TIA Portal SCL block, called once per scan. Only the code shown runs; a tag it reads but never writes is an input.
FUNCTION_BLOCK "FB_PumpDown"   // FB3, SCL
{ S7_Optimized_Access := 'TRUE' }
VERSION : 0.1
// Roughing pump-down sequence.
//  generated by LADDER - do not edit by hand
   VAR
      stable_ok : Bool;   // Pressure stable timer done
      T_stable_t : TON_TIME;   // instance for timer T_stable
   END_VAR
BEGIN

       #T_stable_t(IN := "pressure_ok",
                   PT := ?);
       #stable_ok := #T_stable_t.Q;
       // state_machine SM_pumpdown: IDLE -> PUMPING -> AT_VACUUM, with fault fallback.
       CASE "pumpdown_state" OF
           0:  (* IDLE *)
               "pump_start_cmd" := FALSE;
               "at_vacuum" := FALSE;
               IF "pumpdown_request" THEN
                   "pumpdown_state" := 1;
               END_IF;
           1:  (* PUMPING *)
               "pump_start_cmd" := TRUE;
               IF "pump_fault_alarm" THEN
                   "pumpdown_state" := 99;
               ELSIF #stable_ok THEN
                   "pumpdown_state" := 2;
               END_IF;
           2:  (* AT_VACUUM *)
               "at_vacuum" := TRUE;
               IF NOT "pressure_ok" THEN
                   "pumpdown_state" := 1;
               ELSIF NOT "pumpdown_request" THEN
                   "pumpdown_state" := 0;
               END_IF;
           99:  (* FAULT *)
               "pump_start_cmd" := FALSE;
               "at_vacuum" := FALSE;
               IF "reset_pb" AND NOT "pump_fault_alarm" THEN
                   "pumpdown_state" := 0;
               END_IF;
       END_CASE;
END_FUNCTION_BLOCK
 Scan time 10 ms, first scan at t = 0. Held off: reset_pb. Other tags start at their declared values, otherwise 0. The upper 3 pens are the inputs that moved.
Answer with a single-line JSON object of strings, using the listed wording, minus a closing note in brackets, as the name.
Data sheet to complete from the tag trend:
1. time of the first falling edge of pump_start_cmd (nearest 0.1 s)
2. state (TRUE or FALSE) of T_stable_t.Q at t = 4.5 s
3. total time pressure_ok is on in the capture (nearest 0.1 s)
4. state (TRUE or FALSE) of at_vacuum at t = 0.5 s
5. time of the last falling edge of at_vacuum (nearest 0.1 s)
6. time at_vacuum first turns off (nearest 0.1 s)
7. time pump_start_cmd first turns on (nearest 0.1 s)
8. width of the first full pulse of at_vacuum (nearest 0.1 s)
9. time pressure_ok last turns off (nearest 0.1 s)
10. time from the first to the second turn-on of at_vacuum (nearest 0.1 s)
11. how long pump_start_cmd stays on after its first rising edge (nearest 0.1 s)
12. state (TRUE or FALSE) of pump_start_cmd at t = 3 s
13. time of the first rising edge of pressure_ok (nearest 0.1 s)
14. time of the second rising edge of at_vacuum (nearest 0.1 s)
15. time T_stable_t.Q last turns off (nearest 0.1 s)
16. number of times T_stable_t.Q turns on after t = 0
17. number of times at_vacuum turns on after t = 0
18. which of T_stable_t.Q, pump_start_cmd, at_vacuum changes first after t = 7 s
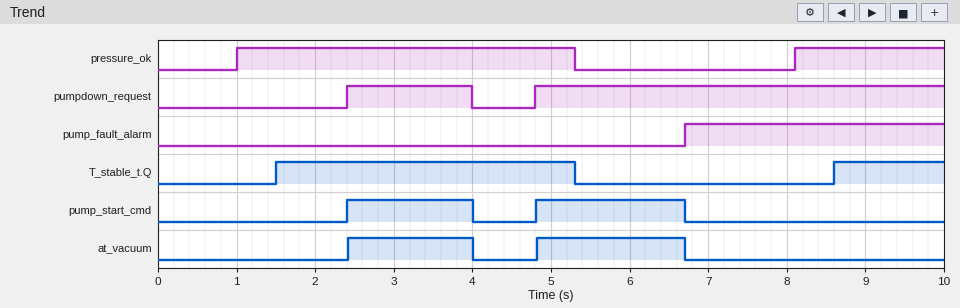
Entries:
{"time of the first falling edge of pump_start_cmd": "4.0 s", "state (TRUE or FALSE) of T_stable_t.Q at t = 4.5 s": "TRUE", "total time pressure_ok is on in the capture": "6.2 s", "state (TRUE or FALSE) of at_vacuum at t = 0.5 s": "FALSE", "time of the last falling edge of at_vacuum": "6.7 s", "time at_vacuum first turns off": "4.0 s", "time pump_start_cmd first turns on": "2.4 s", "width of the first full pulse of at_vacuum": "1.6 s", "time pressure_ok last turns off": "5.3 s", "time from the first to the second turn-on of at_vacuum": "2.4 s", "how long pump_start_cmd stays on after its first rising edge": "1.6 s", "state (TRUE or FALSE) of pump_start_cmd at t = 3 s": "TRUE", "time of the first rising edge of pressure_ok": "1.0 s", "time of the second rising edge of at_vacuum": "4.8 s", "time T_stable_t.Q last turns off": "5.3 s", "number of times T_stable_t.Q turns on after t = 0": "2", "number of times at_vacuum turns on after t = 0": "2", "which of T_stable_t.Q, pump_start_cmd, at_vacuum changes first after t = 7 s": "T_stable_t.Q"}
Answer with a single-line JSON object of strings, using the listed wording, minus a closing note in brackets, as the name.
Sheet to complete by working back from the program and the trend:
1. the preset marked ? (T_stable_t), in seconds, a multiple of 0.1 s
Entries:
{"the preset marked ? (T_stable_t), in seconds, a multiple of 0.1 s": "0.5 s"}
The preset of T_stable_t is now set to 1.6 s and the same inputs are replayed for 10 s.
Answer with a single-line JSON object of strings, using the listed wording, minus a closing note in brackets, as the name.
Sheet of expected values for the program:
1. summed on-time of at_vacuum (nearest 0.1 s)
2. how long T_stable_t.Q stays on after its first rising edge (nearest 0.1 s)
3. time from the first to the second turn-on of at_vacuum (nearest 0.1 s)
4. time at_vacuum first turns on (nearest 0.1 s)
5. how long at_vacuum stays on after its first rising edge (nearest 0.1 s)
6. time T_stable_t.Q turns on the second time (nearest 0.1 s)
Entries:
{"summed on-time of at_vacuum": "3.3 s", "how long T_stable_t.Q stays on after its first rising edge": "2.7 s", "time from the first to the second turn-on of at_vacuum": "2.2 s", "time at_vacuum first turns on": "2.6 s", "how long at_vacuum stays on after its first rising edge": "1.4 s", "time T_stable_t.Q turns on the second time": "9.7 s"}
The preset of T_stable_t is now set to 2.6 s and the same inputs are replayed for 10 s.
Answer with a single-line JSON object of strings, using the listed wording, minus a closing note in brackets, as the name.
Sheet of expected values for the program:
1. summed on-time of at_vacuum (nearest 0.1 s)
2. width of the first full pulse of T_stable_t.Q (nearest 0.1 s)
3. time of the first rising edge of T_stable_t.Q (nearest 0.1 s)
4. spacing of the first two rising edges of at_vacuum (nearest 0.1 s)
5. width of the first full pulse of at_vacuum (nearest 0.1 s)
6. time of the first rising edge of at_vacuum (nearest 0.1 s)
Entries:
{"summed on-time of at_vacuum": "2.3 s", "width of the first full pulse of T_stable_t.Q": "1.7 s", "time of the first rising edge of T_stable_t.Q": "3.6 s", "spacing of the first two rising edges of at_vacuum": "1.2 s", "width of the first full pulse of at_vacuum": "0.4 s", "time of the first rising edge of at_vacuum": "3.6 s"}
